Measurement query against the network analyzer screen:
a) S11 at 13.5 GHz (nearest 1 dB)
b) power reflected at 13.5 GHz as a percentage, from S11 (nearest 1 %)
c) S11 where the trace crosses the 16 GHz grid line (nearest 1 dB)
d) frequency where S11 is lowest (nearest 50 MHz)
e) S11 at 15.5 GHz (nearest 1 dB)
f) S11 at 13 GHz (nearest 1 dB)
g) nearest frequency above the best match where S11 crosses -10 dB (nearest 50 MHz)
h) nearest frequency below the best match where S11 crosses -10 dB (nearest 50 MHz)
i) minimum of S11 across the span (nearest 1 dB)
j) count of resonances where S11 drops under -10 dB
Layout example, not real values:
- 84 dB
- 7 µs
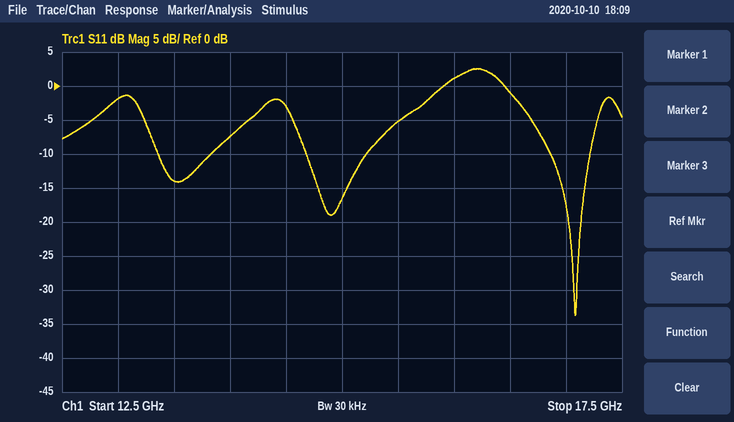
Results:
- -14 dB
- 4 %
- 1 dB
- 17.10 GHz
- -5 dB
- -2 dB
- 17.20 GHz
- 16.85 GHz
- -34 dB
- 3
